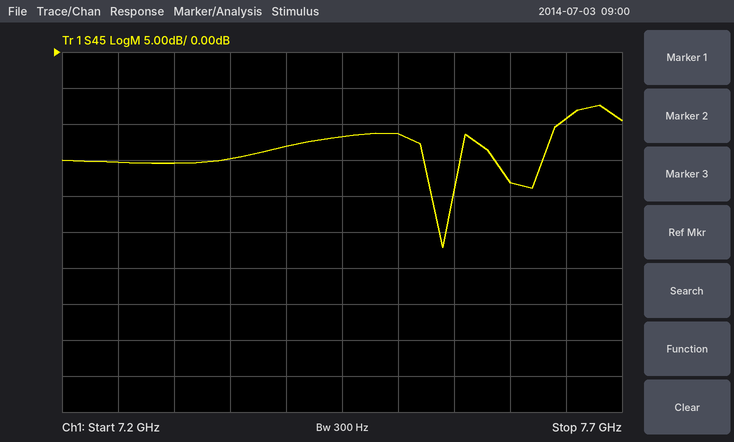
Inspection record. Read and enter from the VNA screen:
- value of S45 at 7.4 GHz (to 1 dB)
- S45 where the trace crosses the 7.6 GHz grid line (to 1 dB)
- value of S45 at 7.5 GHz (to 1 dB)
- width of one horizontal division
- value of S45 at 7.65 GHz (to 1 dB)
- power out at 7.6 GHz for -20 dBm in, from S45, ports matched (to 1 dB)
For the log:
-13 dB
-18 dB
-11 dB
50 MHz
-9 dB
-38 dBm
